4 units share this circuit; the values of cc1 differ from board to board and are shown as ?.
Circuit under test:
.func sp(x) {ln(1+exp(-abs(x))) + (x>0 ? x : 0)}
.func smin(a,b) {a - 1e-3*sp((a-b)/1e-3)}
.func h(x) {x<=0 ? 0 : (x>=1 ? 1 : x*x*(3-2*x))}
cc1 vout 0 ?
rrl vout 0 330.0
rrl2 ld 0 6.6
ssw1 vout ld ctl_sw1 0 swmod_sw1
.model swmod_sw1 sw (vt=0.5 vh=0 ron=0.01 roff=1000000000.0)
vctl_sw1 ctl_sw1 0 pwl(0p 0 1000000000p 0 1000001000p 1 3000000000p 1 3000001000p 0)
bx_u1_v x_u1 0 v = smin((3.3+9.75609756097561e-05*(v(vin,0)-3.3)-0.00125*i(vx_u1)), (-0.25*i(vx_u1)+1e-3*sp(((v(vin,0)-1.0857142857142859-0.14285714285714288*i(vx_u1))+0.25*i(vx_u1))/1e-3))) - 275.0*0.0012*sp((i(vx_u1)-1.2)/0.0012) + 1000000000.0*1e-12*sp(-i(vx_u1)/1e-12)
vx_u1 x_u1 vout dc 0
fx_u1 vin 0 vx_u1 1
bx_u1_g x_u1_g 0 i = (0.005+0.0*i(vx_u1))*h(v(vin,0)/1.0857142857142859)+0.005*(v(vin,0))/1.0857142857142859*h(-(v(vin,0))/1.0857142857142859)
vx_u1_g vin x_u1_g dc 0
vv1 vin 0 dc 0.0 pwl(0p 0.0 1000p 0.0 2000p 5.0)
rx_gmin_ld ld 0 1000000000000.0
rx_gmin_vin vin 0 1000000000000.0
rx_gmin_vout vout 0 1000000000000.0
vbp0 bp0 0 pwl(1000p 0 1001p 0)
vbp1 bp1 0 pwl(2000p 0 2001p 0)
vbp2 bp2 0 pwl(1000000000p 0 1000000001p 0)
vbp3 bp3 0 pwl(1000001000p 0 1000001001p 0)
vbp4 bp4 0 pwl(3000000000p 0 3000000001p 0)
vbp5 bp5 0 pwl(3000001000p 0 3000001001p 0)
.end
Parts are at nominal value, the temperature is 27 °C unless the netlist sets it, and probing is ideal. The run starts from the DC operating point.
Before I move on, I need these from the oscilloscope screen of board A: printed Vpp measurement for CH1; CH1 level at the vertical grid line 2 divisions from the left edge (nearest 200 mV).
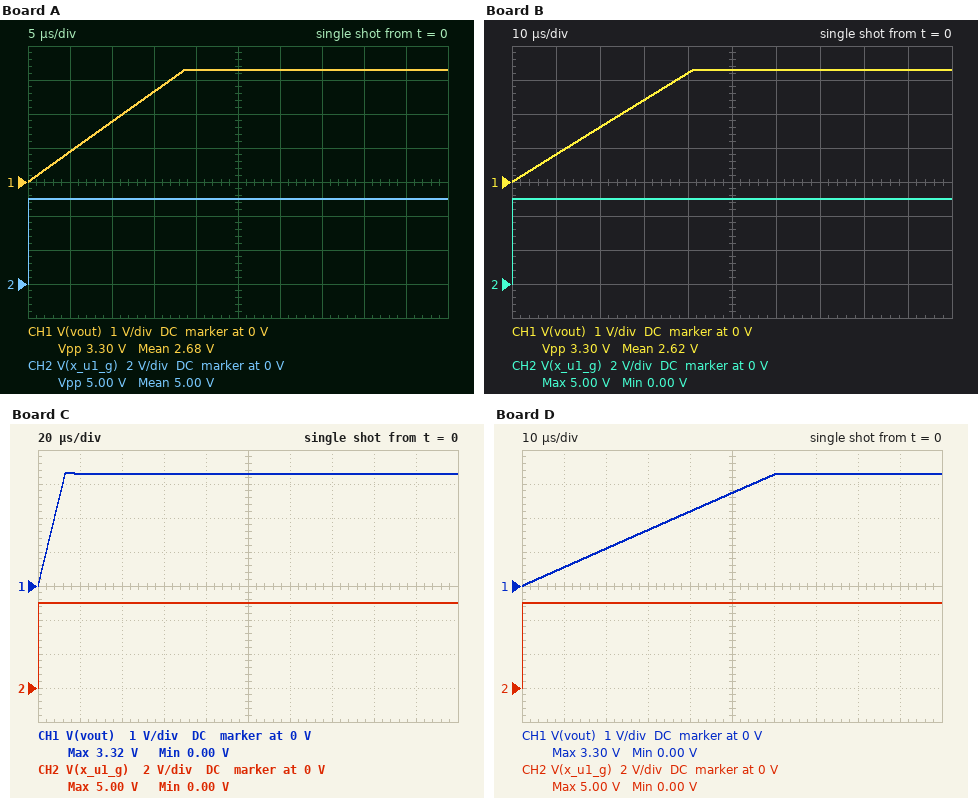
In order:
3.30 V
1.8 V
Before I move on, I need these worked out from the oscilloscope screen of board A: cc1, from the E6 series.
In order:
6.8 µF
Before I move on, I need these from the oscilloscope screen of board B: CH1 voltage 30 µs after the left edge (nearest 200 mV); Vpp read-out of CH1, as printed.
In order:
2.4 V
3.30 V
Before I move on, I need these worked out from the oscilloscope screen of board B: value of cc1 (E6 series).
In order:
15 µF
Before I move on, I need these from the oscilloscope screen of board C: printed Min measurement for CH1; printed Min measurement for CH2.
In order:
0.00 V
0.00 V
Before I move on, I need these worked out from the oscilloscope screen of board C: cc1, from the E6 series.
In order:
4.7 µF
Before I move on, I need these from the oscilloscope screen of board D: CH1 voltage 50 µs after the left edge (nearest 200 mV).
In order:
2.8 V
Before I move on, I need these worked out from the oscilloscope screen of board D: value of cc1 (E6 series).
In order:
22 µF
